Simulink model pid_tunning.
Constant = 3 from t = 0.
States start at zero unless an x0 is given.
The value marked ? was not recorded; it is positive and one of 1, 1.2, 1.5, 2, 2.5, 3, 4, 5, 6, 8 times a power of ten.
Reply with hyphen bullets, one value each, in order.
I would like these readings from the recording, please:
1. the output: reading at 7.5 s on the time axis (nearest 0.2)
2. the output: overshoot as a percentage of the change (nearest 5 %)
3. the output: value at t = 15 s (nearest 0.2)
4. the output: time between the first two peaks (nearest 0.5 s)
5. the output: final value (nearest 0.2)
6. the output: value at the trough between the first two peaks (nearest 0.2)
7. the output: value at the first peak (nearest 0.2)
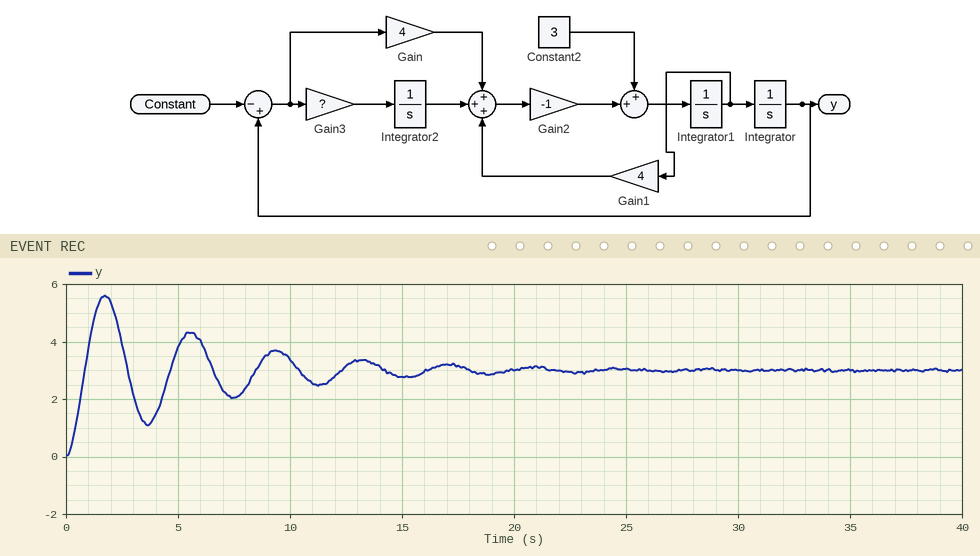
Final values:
- 2.0
- 85 %
- 2.8
- 4.0 s
- 3.0
- 1.2
- 5.6
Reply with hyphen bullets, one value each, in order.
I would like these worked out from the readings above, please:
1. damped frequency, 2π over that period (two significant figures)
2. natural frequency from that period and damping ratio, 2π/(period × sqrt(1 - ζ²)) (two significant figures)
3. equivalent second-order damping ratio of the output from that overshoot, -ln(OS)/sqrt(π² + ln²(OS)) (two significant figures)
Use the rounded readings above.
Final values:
- 1.6 rad/s
- 1.6 rad/s
- 0.052
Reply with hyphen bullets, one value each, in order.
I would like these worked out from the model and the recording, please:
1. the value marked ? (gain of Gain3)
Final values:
- 10
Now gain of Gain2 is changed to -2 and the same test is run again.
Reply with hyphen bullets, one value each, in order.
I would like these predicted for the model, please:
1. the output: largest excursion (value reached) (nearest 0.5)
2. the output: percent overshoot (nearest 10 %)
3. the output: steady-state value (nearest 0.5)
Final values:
- 5.0
- 60 %
- 3.0
